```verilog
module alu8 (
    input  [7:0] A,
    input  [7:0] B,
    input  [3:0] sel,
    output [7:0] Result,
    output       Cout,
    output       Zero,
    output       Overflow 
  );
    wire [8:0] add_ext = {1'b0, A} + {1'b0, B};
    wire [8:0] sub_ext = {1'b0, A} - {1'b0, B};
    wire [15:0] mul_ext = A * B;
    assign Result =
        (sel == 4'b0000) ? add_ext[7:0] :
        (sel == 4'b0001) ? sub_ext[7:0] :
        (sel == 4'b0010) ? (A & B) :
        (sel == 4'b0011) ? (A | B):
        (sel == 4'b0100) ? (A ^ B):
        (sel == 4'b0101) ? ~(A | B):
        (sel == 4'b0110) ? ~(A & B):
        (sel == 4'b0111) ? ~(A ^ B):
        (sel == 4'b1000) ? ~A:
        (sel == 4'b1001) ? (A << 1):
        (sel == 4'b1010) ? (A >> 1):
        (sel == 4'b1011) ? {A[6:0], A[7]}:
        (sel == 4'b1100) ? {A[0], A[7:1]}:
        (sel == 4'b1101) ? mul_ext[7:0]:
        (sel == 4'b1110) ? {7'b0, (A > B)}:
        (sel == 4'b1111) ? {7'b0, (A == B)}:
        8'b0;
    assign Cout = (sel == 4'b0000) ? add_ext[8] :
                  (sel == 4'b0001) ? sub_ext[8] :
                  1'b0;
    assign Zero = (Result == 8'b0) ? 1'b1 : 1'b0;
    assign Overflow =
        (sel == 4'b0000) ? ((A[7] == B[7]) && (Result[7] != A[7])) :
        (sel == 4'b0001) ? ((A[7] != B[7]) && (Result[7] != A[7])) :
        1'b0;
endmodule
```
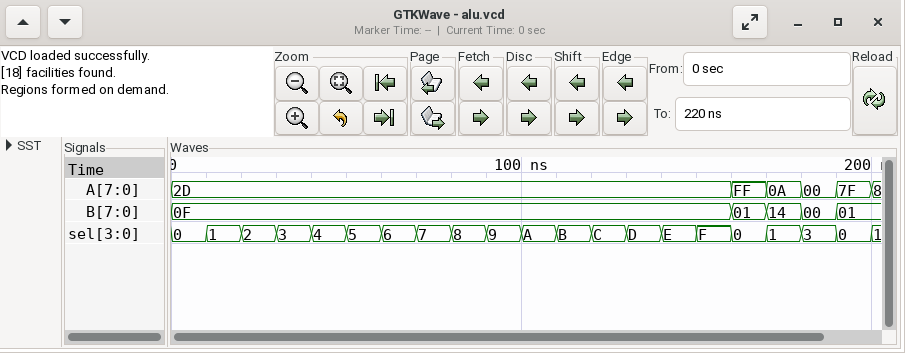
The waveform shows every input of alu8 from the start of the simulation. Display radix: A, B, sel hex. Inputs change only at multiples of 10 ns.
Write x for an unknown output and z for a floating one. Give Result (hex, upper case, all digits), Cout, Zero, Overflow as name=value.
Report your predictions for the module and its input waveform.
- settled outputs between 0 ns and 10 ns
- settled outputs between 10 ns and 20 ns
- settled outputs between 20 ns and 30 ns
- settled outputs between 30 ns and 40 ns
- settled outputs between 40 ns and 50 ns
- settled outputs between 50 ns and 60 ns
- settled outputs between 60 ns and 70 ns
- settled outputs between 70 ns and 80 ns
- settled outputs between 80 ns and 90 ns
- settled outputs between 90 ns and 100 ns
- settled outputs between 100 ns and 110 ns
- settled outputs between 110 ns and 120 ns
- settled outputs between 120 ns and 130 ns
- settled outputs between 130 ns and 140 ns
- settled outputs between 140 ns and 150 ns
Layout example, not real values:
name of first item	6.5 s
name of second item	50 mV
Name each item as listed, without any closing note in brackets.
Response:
settled outputs between 0 ns and 10 ns	Result=3C, Cout=0, Zero=0, Overflow=0
settled outputs between 10 ns and 20 ns	Result=1E, Cout=0, Zero=0, Overflow=0
settled outputs between 20 ns and 30 ns	Result=0D, Cout=0, Zero=0, Overflow=0
settled outputs between 30 ns and 40 ns	Result=2F, Cout=0, Zero=0, Overflow=0
settled outputs between 40 ns and 50 ns	Result=22, Cout=0, Zero=0, Overflow=0
settled outputs between 50 ns and 60 ns	Result=D0, Cout=0, Zero=0, Overflow=0
settled outputs between 60 ns and 70 ns	Result=F2, Cout=0, Zero=0, Overflow=0
settled outputs between 70 ns and 80 ns	Result=DD, Cout=0, Zero=0, Overflow=0
settled outputs between 80 ns and 90 ns	Result=D2, Cout=0, Zero=0, Overflow=0
settled outputs between 90 ns and 100 ns	Result=5A, Cout=0, Zero=0, Overflow=0
settled outputs between 100 ns and 110 ns	Result=16, Cout=0, Zero=0, Overflow=0
settled outputs between 110 ns and 120 ns	Result=5A, Cout=0, Zero=0, Overflow=0
settled outputs between 120 ns and 130 ns	Result=96, Cout=0, Zero=0, Overflow=0
settled outputs between 130 ns and 140 ns	Result=A3, Cout=0, Zero=0, Overflow=0
settled outputs between 140 ns and 150 ns	Result=01, Cout=0, Zero=0, Overflow=0
